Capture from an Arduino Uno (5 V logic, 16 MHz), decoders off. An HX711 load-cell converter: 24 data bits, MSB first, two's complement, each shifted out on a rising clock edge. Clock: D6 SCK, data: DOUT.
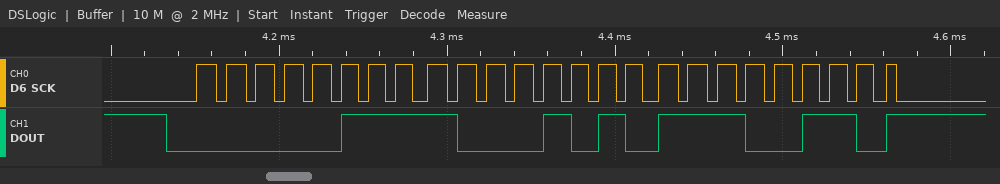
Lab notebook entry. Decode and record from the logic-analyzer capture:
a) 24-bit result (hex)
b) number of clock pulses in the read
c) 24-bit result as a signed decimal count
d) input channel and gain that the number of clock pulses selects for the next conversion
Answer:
0x078AE6
25
494310
channel A, gain 128
